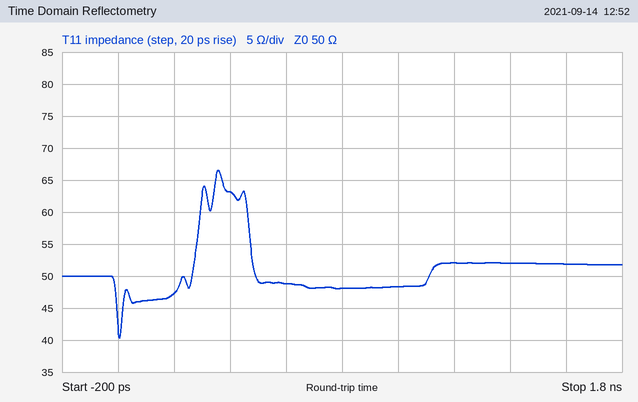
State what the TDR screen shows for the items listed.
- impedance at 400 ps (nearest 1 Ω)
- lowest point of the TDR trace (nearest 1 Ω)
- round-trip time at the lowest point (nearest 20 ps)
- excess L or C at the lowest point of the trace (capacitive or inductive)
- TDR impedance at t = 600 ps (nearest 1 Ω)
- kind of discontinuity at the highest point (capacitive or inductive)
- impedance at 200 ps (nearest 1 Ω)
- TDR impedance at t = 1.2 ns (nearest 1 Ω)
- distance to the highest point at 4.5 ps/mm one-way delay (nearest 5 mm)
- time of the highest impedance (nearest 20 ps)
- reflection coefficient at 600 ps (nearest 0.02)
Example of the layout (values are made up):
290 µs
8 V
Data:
63 Ω
40 Ω
0 ps
capacitive
49 Ω
inductive
47 Ω
52 Ω
40 mm
360 ps
-0.02
